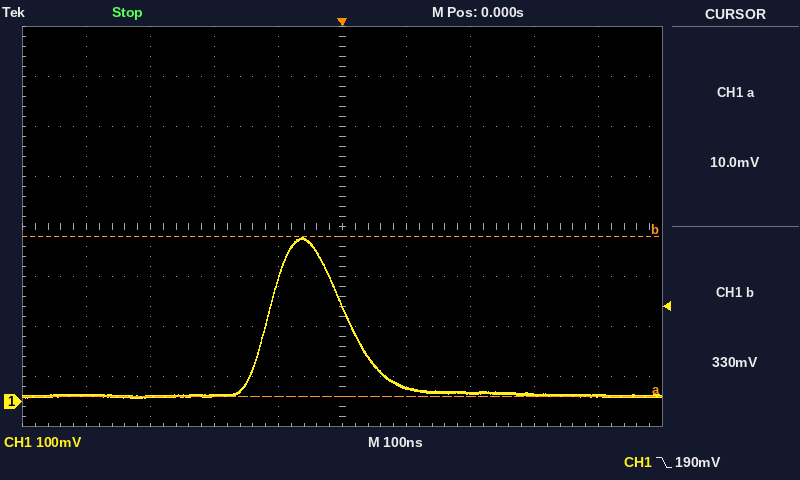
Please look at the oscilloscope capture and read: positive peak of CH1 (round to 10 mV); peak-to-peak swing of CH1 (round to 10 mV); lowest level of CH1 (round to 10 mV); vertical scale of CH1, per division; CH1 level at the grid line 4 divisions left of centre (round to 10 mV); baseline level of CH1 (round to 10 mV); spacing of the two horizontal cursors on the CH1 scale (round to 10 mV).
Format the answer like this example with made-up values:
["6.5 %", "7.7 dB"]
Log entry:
["330 mV", "320 mV", "10 mV", "100 mV", "10 mV", "10 mV", "320 mV"]
